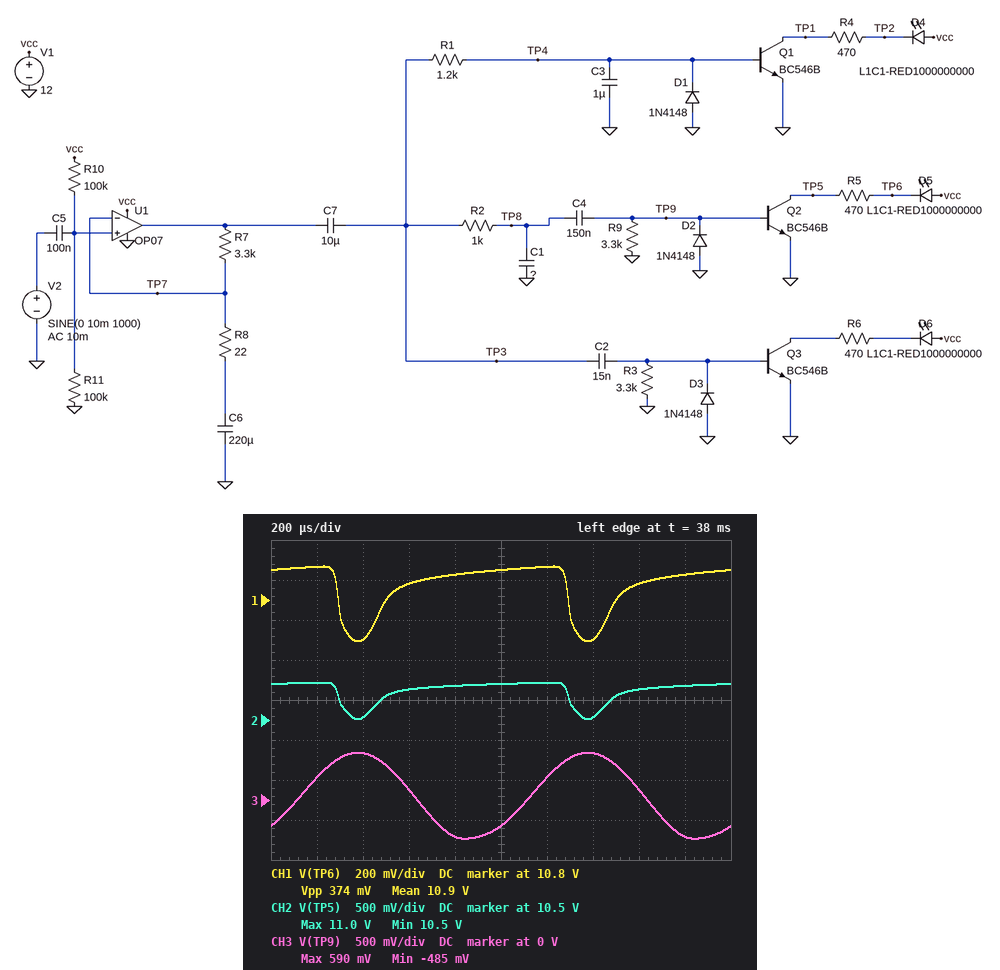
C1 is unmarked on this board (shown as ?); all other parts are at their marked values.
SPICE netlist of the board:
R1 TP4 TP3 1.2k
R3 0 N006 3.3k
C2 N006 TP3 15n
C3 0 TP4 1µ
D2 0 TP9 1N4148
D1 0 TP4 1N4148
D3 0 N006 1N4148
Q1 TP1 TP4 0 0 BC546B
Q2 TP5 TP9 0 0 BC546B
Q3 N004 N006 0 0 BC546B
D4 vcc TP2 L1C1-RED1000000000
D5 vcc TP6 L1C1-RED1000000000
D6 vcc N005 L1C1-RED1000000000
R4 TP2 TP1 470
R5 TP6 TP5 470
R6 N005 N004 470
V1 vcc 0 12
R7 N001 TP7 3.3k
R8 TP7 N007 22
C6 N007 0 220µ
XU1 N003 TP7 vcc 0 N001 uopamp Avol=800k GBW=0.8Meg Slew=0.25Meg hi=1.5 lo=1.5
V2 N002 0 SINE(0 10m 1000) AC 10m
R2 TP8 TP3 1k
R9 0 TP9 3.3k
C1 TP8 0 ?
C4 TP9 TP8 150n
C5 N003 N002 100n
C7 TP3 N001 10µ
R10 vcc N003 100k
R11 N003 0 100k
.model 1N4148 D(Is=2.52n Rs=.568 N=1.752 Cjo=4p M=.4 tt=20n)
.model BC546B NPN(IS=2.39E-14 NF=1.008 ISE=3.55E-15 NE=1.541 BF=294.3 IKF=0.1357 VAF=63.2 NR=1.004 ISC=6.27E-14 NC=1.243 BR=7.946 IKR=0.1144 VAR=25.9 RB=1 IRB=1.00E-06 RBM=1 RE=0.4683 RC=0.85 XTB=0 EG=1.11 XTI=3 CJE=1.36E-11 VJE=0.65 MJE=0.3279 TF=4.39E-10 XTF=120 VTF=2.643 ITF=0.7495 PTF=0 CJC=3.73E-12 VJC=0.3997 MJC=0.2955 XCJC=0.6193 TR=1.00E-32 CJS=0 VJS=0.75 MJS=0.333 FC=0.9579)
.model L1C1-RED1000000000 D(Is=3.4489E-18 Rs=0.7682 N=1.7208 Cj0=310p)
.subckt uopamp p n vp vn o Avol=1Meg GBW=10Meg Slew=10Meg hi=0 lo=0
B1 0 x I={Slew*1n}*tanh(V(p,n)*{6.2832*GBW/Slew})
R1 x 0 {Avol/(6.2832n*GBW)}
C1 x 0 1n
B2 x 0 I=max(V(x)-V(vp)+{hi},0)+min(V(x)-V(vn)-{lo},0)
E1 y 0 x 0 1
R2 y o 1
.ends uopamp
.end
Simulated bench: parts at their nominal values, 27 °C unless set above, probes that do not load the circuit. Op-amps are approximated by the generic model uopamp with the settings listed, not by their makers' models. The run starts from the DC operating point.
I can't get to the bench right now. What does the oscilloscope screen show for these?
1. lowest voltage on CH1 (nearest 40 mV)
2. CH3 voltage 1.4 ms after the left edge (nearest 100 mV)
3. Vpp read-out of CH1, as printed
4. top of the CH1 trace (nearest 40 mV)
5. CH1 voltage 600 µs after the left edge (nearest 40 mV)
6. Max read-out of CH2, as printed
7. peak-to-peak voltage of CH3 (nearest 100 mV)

10.60 V
600 mV
374 mV
10.96 V
10.88 V
11.0 V
1.1 V
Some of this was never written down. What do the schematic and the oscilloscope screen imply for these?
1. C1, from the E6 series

330 nF
